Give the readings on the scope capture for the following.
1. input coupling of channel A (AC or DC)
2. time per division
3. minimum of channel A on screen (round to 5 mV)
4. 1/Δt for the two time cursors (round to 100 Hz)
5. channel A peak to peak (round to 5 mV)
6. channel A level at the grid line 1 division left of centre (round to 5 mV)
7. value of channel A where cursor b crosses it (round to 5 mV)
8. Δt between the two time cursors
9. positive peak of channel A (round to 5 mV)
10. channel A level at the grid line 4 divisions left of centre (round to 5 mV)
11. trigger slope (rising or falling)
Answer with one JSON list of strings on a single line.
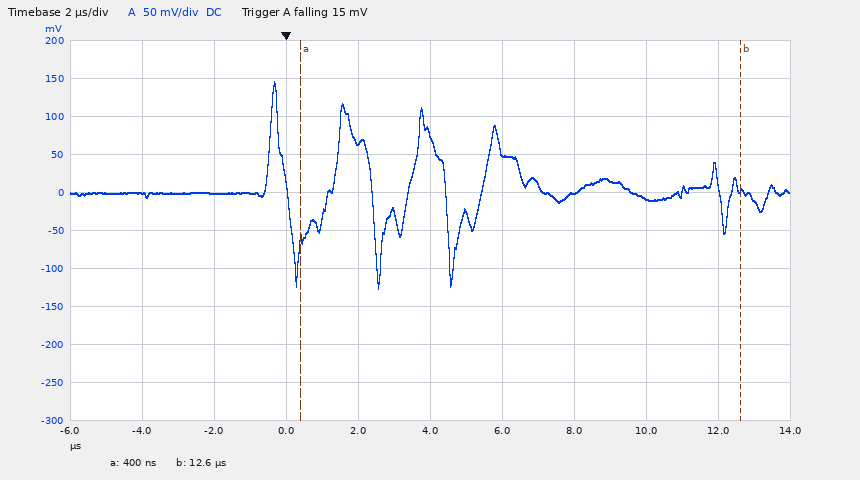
["DC", "2 µs", "-125 mV", "82.0 kHz", "270 mV", "65 mV", "5 mV", "12.2 µs", "145 mV", "0 mV", "falling"]
